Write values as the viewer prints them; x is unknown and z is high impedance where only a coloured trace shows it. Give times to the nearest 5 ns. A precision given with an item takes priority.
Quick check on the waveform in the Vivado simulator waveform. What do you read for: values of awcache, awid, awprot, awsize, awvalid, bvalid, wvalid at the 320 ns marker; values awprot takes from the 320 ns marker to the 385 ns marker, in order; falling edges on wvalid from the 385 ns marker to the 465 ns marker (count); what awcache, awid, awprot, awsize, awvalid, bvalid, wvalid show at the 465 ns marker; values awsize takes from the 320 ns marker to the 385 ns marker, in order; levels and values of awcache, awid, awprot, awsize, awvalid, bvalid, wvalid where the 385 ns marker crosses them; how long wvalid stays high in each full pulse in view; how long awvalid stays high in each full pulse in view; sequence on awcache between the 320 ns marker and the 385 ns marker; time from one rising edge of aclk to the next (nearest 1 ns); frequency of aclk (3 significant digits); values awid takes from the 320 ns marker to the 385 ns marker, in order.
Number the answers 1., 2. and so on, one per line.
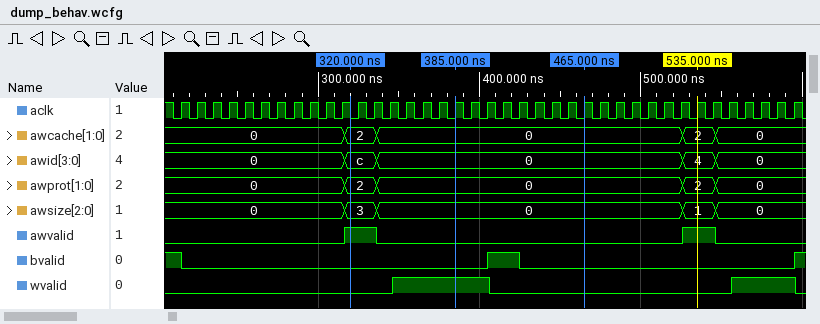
1. awcache=2, awid=c, awprot=2, awsize=3, awvalid=1, bvalid=0, wvalid=0
2. 2, 0
3. 1
4. awcache=0, awid=0, awprot=0, awsize=0, awvalid=0, bvalid=0, wvalid=0
5. 3, 0
6. awcache=0, awid=0, awprot=0, awsize=0, awvalid=0, bvalid=0, wvalid=1
7. 60 ns, 40 ns
8. 20 ns, 20 ns
9. 2, 0
10. 10 ns
11. 100 MHz
12. c, 0
